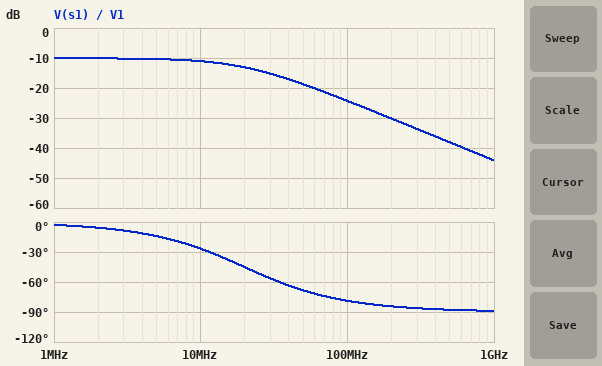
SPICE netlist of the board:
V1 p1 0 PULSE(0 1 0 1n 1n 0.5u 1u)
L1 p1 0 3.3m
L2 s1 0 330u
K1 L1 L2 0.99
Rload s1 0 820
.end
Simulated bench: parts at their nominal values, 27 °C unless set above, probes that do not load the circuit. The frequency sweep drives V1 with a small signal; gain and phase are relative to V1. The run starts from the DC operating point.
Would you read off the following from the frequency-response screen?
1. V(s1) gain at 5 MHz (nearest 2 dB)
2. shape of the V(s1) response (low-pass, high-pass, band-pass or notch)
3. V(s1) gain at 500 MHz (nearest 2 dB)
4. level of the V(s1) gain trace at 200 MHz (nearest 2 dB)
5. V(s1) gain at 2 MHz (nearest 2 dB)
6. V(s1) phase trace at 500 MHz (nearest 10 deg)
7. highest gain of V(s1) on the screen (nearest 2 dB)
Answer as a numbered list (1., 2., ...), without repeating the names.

1. -10 dB
2. low-pass
3. -38 dB
4. -30 dB
5. -10 dB
6. -90 deg
7. -10 dB
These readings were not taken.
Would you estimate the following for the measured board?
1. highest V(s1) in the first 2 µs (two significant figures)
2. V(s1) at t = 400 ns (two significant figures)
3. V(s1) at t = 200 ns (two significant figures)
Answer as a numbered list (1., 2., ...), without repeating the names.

1. 310 mV
2. 310 mV
3. 310 mV
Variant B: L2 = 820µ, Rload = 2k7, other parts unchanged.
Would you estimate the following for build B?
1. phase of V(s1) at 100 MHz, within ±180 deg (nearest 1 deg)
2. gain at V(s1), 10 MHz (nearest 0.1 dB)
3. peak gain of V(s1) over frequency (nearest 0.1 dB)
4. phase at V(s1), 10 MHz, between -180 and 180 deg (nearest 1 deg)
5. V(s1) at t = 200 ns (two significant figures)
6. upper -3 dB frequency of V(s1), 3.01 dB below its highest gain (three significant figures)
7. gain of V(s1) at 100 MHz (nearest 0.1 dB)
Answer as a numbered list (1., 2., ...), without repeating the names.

1. -75 deg
2. -6.7 dB
3. -6.1 dB
4. -21 deg
5. 490 mV
6. 26.3 MHz
7. -18.0 dB
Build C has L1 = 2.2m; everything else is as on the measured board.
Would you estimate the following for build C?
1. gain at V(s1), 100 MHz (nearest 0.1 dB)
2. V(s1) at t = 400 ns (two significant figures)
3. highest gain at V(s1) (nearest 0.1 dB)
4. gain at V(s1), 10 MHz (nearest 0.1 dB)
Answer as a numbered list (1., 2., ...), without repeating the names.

1. -22.5 dB
2. 380 mV
3. -8.3 dB
4. -9.3 dB
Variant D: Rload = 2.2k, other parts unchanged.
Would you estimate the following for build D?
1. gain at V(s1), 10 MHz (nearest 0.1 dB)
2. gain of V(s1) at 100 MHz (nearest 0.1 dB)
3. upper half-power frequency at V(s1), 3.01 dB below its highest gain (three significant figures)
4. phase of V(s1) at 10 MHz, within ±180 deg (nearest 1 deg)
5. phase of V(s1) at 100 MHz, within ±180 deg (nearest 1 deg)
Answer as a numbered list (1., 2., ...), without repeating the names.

1. -10.2 dB
2. -16.6 dB
3. 53.3 MHz
4. -11 deg
5. -62 deg
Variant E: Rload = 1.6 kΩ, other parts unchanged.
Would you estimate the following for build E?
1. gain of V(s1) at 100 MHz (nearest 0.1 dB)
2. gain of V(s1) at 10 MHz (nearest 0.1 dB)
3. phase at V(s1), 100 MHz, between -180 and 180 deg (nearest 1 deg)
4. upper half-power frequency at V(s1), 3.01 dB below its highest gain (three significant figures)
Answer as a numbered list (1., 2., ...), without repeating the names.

1. -18.9 dB
2. -10.4 dB
3. -69 deg
4. 38.8 MHz
